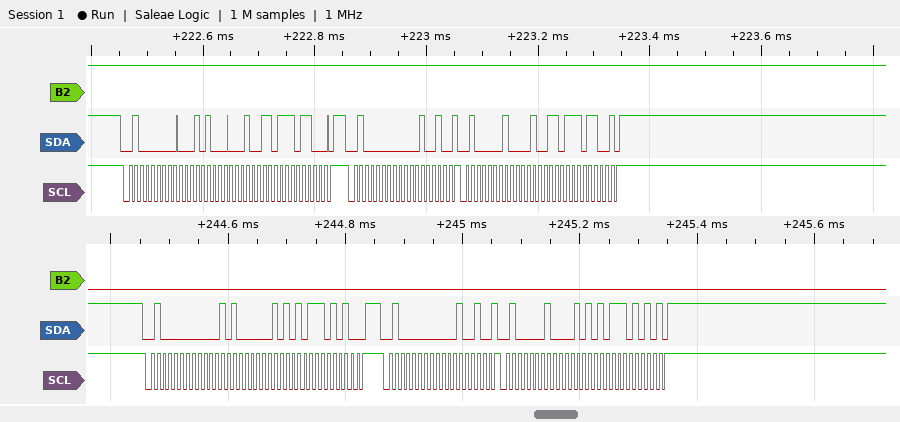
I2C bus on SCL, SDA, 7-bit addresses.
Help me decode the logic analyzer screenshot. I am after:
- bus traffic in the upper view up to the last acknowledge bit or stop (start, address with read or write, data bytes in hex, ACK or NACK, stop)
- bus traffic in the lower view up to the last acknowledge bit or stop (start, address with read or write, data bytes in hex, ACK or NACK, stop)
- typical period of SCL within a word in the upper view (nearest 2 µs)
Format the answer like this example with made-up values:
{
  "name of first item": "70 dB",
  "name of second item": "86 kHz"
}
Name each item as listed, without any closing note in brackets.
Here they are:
{
  "bus traffic in the upper view up to the last acknowledge bit or stop": "start, address 20 write ACK, 14 ACK, 13 ACK, EC ACK, stop, start, address 20 write ACK, 12 ACK, repeated start, address 20 read ACK, 13 ACK, EC NACK, stop",
  "bus traffic in the lower view up to the last acknowledge bit or stop": "start, address 20 write ACK, 14 ACK, 15 ACK, EA ACK, stop, start, address 20 write ACK, 12 ACK, repeated start, address 20 read ACK, 15 ACK, EA NACK, stop",
  "typical period of SCL within a word in the upper view": "10 µs"
}
